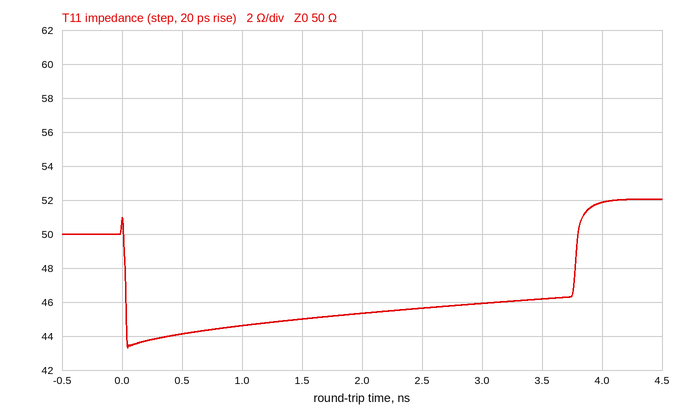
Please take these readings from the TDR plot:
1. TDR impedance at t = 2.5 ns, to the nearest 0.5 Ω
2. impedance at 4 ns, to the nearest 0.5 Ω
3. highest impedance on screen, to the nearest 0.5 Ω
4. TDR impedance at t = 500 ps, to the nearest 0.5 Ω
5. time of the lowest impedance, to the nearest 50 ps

45.5 Ω
52.0 Ω
52.0 Ω
44.0 Ω
50 ps
